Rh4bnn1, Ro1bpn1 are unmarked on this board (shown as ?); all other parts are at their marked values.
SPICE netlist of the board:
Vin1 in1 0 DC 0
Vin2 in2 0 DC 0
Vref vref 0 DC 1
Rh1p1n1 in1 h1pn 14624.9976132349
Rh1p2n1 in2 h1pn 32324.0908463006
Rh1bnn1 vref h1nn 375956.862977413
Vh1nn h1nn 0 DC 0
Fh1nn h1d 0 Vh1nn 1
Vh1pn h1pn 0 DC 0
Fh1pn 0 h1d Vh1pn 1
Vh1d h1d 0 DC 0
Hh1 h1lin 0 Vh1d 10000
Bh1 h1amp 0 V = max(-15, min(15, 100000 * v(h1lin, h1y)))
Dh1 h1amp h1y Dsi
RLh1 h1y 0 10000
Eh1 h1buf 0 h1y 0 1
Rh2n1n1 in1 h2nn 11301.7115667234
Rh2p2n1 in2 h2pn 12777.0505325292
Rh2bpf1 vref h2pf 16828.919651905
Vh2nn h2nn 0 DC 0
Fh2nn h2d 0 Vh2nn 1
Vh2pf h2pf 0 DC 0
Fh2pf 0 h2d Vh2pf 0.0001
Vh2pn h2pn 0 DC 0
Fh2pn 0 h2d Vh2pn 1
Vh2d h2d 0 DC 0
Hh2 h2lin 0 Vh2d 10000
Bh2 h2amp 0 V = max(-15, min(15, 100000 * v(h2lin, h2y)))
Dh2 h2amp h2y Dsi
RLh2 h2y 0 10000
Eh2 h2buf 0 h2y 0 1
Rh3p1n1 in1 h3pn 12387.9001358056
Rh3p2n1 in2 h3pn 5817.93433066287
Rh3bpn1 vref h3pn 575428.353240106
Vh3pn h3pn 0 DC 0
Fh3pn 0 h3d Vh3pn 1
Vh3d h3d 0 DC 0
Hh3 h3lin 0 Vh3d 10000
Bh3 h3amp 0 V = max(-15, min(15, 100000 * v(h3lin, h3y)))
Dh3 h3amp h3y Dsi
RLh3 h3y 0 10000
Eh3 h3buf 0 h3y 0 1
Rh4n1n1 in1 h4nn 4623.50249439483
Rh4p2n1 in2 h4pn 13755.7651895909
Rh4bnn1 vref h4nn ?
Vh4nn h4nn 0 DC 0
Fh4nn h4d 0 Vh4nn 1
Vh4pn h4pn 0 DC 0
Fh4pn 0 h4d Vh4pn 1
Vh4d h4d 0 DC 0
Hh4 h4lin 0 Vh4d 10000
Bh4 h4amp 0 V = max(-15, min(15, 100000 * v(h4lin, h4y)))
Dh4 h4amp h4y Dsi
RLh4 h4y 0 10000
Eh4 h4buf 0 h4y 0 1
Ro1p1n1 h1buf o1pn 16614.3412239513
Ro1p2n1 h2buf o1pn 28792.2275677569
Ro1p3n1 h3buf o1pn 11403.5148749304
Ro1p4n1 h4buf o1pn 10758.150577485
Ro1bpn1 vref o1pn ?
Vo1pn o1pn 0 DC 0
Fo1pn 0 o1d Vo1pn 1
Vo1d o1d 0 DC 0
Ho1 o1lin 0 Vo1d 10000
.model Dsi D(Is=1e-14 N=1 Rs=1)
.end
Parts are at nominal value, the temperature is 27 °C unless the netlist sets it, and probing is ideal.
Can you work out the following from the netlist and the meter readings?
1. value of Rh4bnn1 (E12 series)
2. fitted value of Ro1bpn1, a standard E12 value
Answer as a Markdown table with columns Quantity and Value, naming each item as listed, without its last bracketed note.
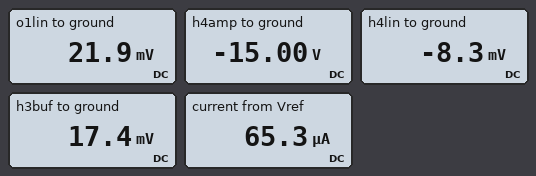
| Quantity | Value |
|---|---|
| value of Rh4bnn1 | 1.2 MΩ |
| fitted value of Ro1bpn1, a standard E12 value | 1.5 MΩ |
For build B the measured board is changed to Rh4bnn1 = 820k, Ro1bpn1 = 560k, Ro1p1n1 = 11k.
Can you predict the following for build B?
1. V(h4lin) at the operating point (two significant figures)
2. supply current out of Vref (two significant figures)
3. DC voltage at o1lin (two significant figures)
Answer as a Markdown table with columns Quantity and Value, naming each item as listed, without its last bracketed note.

| Quantity | Value |
|---|---|
| V(h4lin) at the operating point | -12 mV |
| supply current out of Vref | 67 µA |
| DC voltage at o1lin | 33 mV |
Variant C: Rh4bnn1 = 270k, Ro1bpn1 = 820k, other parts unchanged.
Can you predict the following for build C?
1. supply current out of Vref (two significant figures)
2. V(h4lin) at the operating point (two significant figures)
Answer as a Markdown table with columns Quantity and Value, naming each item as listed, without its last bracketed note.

| Quantity | Value |
|---|---|
| supply current out of Vref | 69 µA |
| V(h4lin) at the operating point | -37 mV |
